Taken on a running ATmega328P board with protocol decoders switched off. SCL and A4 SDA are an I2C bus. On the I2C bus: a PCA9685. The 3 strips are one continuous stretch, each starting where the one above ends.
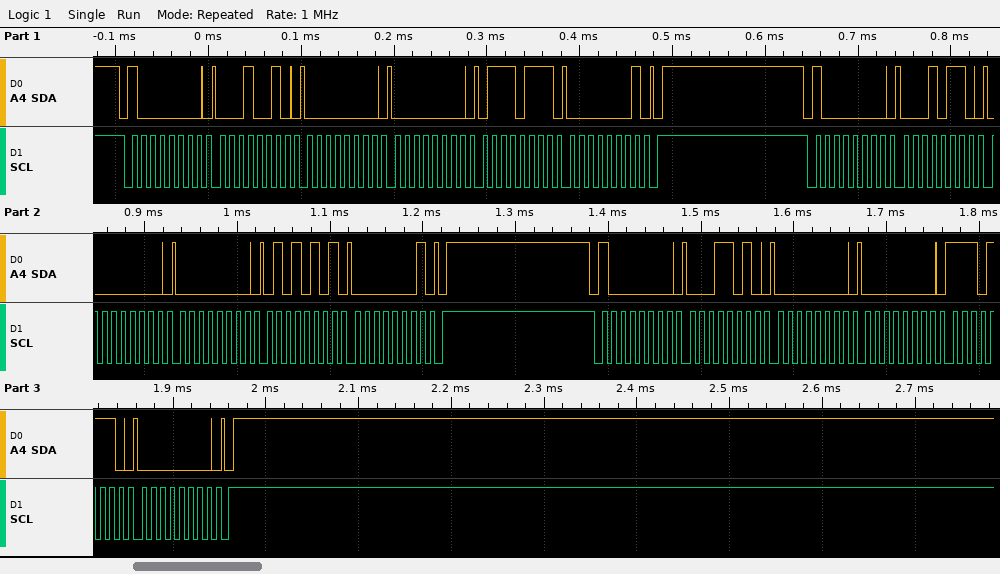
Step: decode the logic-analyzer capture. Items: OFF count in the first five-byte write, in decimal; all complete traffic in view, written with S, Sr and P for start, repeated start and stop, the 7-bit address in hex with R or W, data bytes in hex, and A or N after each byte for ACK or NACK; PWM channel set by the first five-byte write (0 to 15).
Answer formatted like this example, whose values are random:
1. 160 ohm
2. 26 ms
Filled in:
1. 375
2. S 40W A 12 A 00 A 00 A 77 A 01 A P S 40W A 16 A 00 A 00 A 55 A 01 A P S 40W A 1A A 00 A 00 A EE A 00 A P
3. 3
